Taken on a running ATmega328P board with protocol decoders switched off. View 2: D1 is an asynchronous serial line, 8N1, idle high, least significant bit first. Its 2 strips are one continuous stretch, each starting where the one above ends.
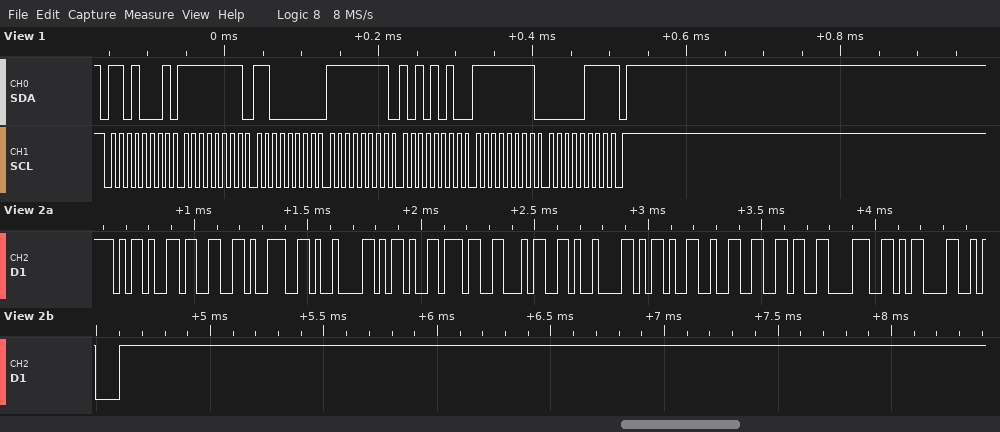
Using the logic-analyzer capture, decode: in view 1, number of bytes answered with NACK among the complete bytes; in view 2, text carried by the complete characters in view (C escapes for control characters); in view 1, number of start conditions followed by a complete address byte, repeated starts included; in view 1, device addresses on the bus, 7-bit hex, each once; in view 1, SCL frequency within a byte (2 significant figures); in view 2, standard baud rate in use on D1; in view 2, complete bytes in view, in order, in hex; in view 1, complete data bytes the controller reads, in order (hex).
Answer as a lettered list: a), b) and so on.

a) 1
b) "-39\t-74\t-268\r\n"
c) 1
d) 0x68
e) 100 kHz
f) 38400 baud
g) 2D 33 39 09 2D 37 34 09 2D 32 36 38 0D 0A
h) FF C0 FF AA FF 07
